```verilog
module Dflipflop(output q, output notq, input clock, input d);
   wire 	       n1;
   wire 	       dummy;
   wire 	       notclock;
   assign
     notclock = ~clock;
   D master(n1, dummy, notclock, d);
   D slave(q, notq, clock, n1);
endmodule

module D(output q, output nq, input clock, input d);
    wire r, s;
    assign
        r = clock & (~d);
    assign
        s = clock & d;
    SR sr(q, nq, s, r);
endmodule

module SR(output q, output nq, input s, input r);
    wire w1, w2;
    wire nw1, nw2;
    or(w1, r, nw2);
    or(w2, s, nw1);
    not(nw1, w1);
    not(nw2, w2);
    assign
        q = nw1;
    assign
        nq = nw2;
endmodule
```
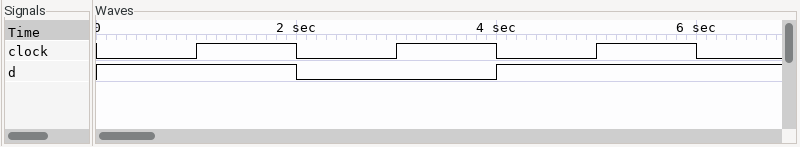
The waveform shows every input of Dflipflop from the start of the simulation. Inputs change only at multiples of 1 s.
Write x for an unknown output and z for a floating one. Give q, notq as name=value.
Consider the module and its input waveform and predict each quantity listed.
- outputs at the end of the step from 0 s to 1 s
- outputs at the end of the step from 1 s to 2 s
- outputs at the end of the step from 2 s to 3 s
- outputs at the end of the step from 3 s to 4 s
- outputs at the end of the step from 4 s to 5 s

q=x, notq=x
q=1, notq=0
q=1, notq=0
q=0, notq=1
q=0, notq=1
